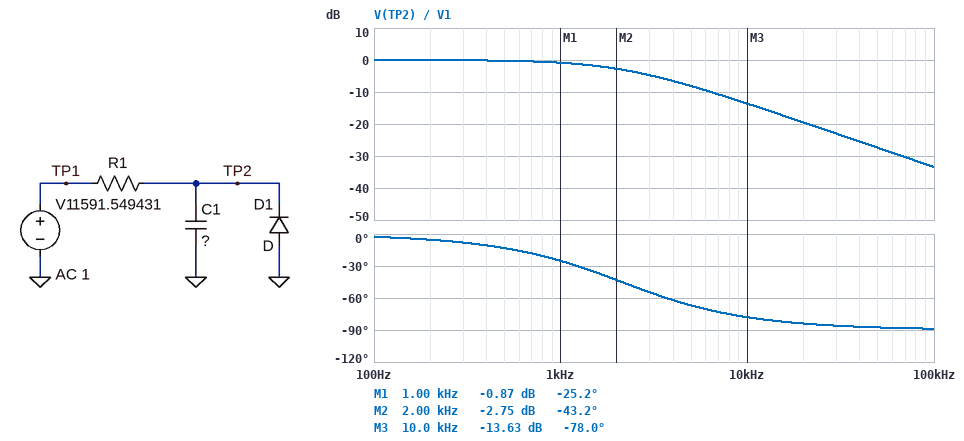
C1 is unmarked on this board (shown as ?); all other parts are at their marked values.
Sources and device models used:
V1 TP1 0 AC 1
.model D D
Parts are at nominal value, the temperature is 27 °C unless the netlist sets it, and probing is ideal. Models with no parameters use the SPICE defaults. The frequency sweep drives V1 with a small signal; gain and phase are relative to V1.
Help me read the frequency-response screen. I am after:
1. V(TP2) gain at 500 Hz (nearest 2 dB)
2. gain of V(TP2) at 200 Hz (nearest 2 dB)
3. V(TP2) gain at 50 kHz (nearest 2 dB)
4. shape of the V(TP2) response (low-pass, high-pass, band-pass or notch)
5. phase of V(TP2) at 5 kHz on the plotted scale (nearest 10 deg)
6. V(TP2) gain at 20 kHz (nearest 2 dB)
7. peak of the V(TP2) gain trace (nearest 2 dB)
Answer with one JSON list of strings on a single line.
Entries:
["0 dB", "0 dB", "-28 dB", "low-pass", "-70 deg", "-20 dB", "0 dB"]
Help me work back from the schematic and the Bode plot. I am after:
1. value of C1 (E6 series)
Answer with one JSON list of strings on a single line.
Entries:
["47 nF"]
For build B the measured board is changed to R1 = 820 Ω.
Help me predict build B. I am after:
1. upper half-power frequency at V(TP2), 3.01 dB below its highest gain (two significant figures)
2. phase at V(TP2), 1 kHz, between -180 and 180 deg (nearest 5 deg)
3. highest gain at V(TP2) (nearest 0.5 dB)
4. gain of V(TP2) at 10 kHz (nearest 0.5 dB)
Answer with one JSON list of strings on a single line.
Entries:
["4.1 kHz", "-15 deg", "0 dB", "-8.5 dB"]
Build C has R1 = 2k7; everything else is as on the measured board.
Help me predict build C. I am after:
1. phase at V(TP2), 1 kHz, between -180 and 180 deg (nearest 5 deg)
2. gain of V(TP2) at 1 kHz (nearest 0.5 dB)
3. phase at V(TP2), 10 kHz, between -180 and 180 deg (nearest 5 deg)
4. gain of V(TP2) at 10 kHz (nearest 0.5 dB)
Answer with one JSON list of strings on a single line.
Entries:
["-40 deg", "-2.0 dB", "-85 deg", "-18.0 dB"]
